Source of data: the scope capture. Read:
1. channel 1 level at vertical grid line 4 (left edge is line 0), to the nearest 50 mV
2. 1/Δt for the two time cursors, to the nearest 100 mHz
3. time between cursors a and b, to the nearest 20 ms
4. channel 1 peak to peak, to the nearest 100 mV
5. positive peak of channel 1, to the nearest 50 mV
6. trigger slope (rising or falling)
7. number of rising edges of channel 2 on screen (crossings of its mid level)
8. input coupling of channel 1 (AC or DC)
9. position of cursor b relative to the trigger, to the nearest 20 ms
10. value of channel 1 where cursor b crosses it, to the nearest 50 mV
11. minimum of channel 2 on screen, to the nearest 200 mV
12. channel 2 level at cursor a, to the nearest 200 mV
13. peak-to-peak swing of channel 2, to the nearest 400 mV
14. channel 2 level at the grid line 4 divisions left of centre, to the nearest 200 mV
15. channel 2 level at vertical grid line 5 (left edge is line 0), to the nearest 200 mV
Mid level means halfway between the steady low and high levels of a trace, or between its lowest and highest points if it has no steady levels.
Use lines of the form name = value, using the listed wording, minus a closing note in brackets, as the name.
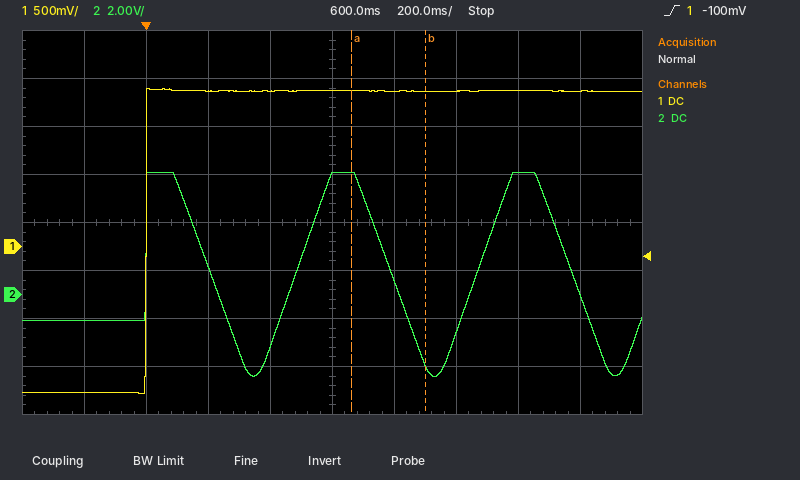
channel 1 level at vertical grid line 4 (left edge is line 0), to the nearest 50 mV = 1.60 V
1/Δt for the two time cursors, to the nearest 100 mHz = 4.2 Hz
time between cursors a and b, to the nearest 20 ms = 240 ms
channel 1 peak to peak, to the nearest 100 mV = 3.20 V
positive peak of channel 1, to the nearest 50 mV = 1.65 V
trigger slope = rising
number of rising edges of channel 2 on screen = 3
input coupling of channel 1 = DC
position of cursor b relative to the trigger, to the nearest 20 ms = +900 ms
value of channel 1 where cursor b crosses it, to the nearest 50 mV = 1.60 V
minimum of channel 2 on screen, to the nearest 200 mV = -3.4 V
channel 2 level at cursor a, to the nearest 200 mV = 5.0 V
peak-to-peak swing of channel 2, to the nearest 400 mV = 8.4 V
channel 2 level at the grid line 4 divisions left of centre, to the nearest 200 mV = -1.0 V
channel 2 level at vertical grid line 5 (left edge is line 0), to the nearest 200 mV = 5.0 V
